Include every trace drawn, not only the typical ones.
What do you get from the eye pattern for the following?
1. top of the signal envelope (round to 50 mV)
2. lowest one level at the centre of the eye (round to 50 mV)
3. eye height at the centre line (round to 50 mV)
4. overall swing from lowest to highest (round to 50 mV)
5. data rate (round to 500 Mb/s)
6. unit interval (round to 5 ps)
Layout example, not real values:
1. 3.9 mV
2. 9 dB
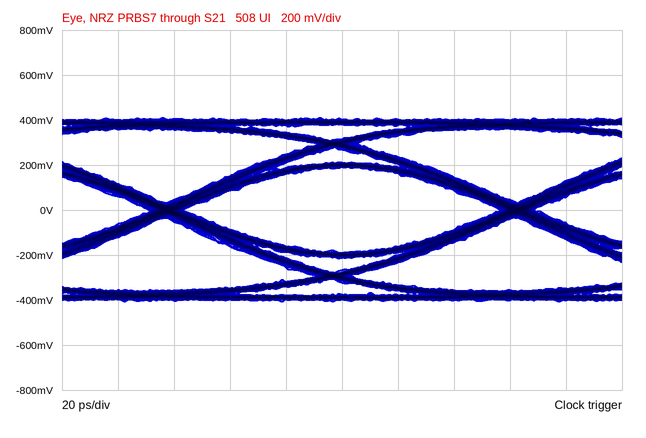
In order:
1. 400 mV
2. 200 mV
3. 400 mV
4. 800 mV
5. 8.0 Gb/s
6. 125 ps
